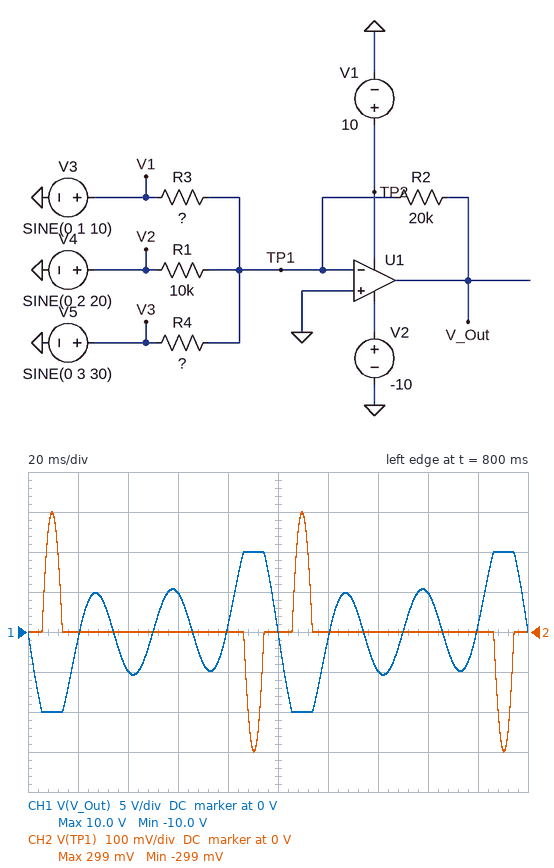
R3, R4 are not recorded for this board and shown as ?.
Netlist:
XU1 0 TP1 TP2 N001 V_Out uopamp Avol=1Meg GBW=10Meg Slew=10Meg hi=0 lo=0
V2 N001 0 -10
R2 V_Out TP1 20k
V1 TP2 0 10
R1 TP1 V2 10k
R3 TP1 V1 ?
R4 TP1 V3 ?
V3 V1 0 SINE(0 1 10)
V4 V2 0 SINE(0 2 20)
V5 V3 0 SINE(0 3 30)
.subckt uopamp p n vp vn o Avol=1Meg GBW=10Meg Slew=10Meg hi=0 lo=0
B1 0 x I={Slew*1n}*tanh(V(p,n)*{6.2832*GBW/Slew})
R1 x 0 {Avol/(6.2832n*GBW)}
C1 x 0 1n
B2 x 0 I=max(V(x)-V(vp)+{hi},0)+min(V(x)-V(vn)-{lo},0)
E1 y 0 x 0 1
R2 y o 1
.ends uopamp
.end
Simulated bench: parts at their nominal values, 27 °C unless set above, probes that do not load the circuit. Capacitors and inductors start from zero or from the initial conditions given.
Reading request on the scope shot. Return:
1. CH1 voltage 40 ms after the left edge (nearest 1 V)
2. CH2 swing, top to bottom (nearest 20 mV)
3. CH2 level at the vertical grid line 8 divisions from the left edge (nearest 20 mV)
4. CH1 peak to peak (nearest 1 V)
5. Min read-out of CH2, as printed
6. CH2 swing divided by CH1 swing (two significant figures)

-5 V
600 mV
0 V
20 V
-299 mV
0.030
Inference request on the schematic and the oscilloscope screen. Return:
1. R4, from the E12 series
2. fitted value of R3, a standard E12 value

8.2 kΩ
6.8 kΩ
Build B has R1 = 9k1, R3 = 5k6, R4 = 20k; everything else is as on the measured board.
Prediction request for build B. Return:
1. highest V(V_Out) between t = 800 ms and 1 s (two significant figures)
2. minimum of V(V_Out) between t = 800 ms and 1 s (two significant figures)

9.2 V
-9.2 V
